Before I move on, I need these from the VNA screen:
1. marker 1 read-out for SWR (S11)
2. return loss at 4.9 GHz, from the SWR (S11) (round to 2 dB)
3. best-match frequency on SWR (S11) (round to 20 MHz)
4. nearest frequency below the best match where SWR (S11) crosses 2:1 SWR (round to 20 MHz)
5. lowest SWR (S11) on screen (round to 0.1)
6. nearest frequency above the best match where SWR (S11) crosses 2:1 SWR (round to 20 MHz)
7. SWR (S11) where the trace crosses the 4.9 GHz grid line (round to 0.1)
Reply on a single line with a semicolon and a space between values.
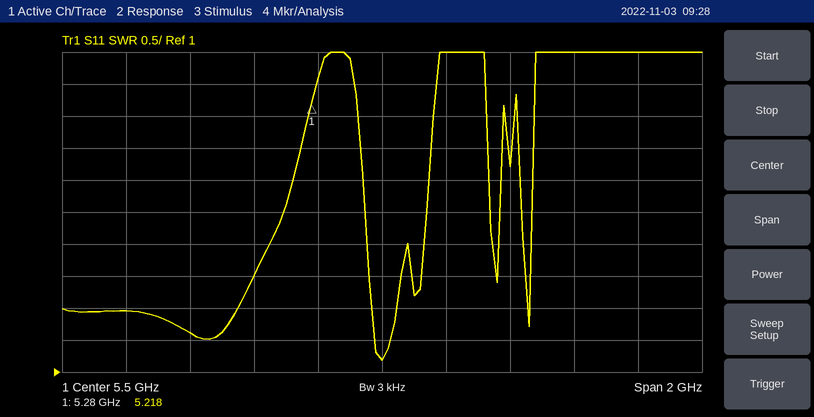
5.218; 12 dB; 5.50 GHz; 5.46 GHz; 1.2; 5.54 GHz; 1.6
